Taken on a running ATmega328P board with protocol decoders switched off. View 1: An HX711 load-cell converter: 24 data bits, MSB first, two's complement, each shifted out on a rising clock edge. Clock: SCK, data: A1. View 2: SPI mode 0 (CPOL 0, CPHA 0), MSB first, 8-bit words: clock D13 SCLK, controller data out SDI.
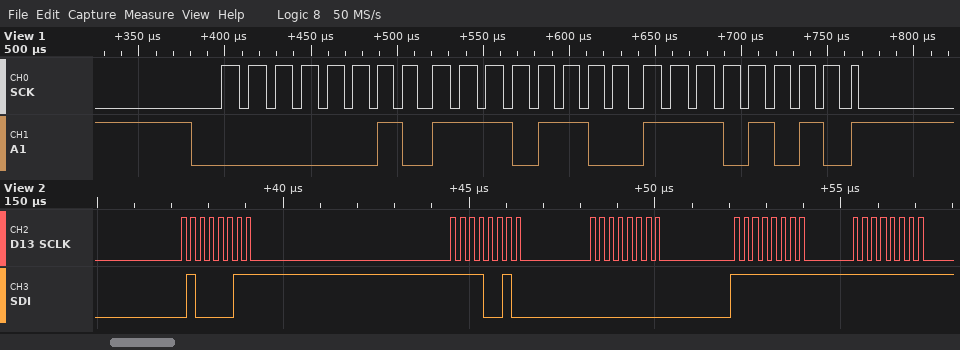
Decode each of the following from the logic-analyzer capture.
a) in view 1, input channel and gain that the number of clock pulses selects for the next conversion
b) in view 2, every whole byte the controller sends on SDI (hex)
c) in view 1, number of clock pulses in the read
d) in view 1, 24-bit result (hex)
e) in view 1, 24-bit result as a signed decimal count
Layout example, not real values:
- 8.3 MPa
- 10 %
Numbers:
- channel A, gain 128
- 43 F2 00 FF FF
- 25
- 0x02ECEA
- 191722
